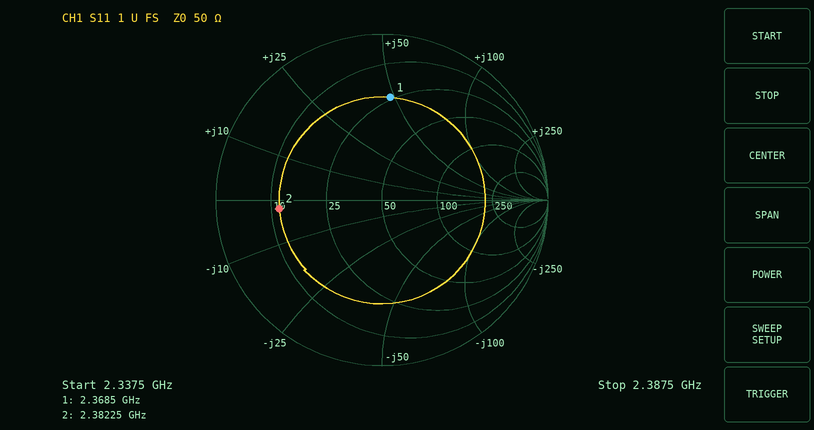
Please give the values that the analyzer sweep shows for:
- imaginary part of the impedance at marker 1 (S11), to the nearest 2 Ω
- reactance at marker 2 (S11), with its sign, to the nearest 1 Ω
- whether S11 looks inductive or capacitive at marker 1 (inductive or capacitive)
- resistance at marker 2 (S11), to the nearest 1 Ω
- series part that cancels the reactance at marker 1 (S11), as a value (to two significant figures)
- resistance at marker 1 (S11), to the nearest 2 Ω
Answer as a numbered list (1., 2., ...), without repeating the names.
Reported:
1. +48 Ω
2. -2 Ω
3. inductive
4. 12 Ω
5. 1.4 pF
6. 24 Ω
